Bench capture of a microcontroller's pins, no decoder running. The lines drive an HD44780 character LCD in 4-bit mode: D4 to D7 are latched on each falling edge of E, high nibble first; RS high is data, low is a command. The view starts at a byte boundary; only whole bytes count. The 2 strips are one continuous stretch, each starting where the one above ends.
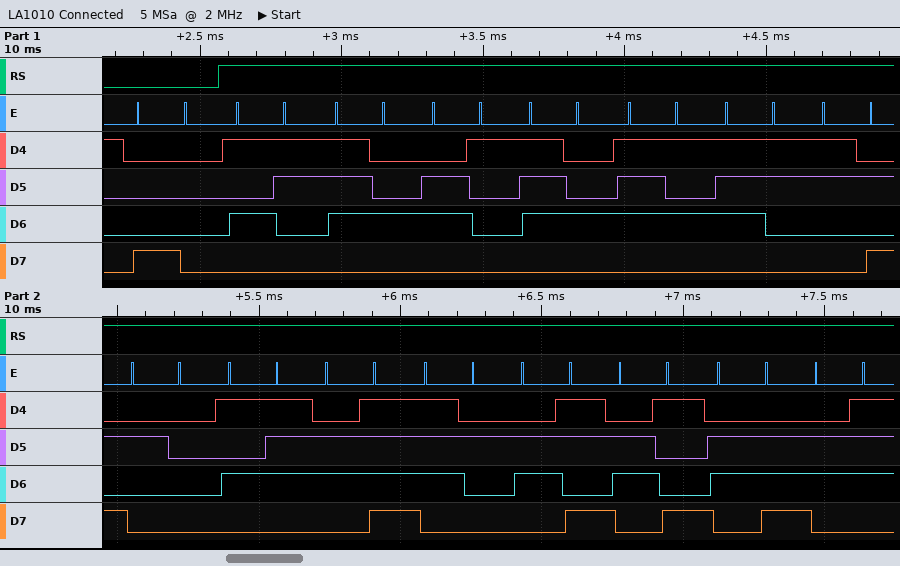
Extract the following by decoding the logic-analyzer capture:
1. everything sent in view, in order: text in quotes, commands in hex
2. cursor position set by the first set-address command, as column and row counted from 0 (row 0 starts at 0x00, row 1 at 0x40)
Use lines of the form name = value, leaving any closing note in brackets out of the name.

everything sent in view, in order: text in quotes, commands in hex = 0x80 "Status: Working"
cursor position set by the first set-address command, as column and row counted from 0 = column 0, row 0
